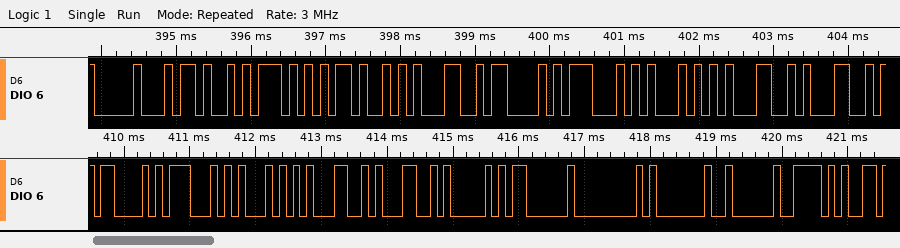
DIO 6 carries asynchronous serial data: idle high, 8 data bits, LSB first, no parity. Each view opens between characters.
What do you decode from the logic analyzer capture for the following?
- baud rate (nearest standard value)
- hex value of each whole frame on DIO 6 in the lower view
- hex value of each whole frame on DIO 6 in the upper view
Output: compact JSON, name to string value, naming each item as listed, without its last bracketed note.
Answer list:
{"baud rate": "9600 baud", "hex value of each whole frame on DIO 6 in the lower view": "43, 47, 51, 31, 31, 41, 03, 00, 01, 02, 5E", "hex value of each whole frame on DIO 6 in the upper view": "10, 4B, 57, 4B, 31, 43, 47, 51, 31, 31"}
